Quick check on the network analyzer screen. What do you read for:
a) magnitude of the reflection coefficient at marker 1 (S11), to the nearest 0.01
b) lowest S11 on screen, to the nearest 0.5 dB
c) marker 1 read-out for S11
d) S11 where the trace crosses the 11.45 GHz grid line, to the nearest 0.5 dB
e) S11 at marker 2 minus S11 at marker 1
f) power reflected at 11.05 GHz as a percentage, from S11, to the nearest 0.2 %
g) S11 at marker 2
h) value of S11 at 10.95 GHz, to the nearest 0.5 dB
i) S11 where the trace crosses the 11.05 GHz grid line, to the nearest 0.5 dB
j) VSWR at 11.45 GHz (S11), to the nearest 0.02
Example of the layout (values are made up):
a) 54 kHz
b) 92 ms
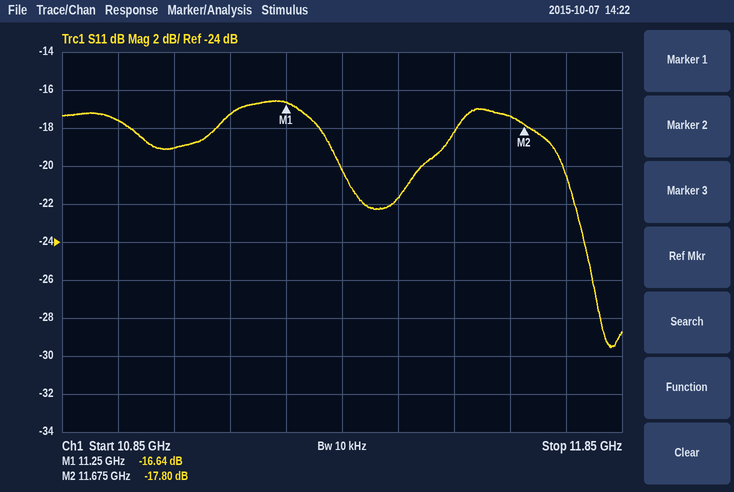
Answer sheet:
a) 0.15
b) -29.5 dB
c) -16.64 dB
d) -21.5 dB
e) -1.16 dB
f) 1.2 %
g) -17.80 dB
h) -17.5 dB
i) -19.0 dB
j) 1.18
